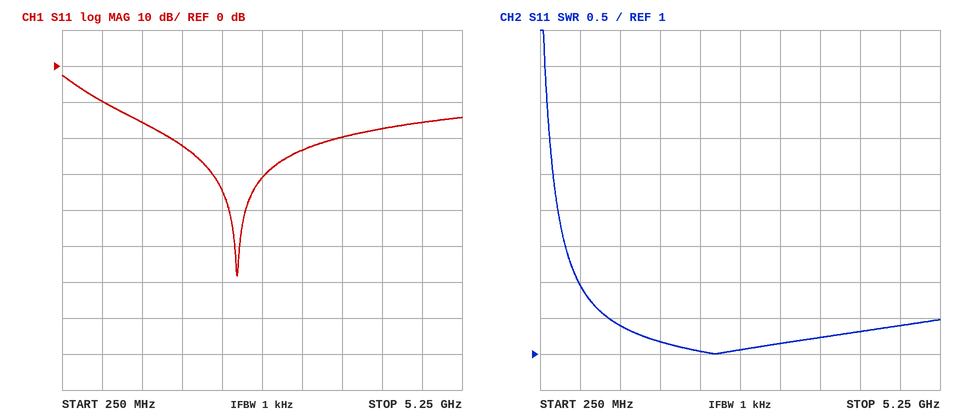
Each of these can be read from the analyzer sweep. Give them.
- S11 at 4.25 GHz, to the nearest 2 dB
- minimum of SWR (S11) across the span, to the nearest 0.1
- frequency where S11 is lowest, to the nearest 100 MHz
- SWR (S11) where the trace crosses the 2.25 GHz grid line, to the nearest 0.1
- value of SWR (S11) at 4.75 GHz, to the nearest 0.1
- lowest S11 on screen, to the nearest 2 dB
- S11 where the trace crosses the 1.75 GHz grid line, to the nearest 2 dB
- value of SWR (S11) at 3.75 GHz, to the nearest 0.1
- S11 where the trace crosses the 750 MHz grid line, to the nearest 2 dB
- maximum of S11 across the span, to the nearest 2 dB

-18 dB
1.0
2.4 GHz
1.0
1.4
-58 dB
-22 dB
1.2
-10 dB
-2 dB
